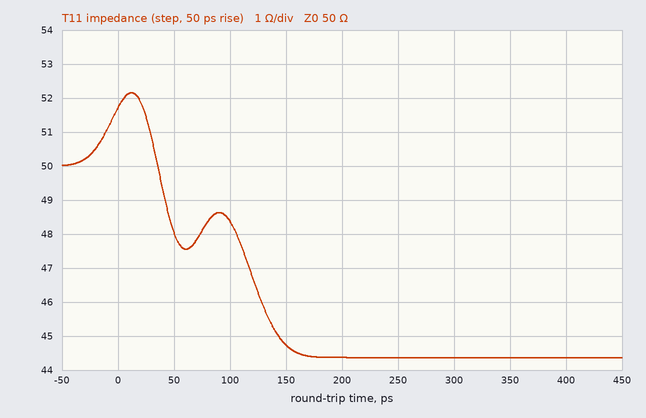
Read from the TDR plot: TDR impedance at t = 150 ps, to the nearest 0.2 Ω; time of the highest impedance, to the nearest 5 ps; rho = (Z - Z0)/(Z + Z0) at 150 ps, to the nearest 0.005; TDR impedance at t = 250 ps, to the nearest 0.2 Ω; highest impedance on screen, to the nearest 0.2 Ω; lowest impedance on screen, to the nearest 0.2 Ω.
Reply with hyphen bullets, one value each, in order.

- 44.8 Ω
- 10 ps
- -0.055
- 44.4 Ω
- 52.2 Ω
- 44.4 Ω
